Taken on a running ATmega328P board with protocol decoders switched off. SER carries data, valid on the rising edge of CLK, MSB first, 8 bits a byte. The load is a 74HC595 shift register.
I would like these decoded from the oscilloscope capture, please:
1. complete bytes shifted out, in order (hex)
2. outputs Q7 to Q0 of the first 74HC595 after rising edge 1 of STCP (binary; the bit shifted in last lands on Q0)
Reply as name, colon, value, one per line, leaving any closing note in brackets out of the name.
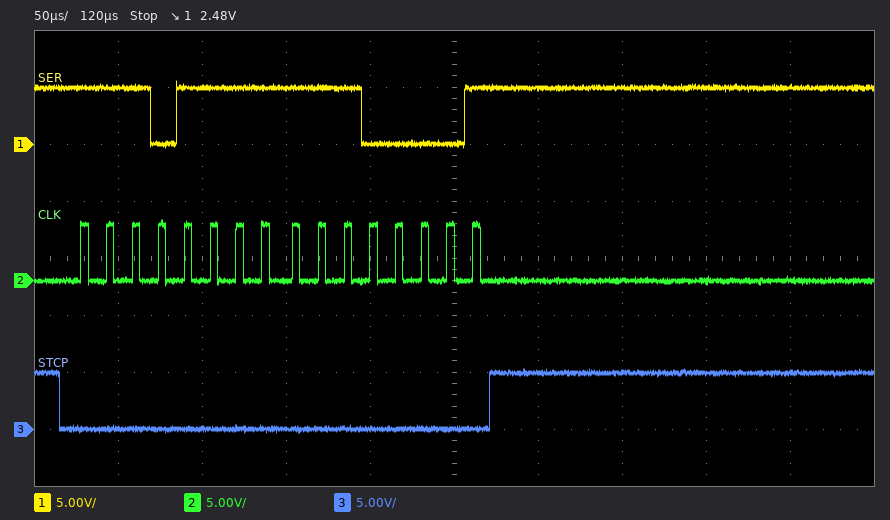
complete bytes shifted out, in order: EF E1
outputs Q7 to Q0 of the first 74HC595 after rising edge 1 of STCP: 11100001
